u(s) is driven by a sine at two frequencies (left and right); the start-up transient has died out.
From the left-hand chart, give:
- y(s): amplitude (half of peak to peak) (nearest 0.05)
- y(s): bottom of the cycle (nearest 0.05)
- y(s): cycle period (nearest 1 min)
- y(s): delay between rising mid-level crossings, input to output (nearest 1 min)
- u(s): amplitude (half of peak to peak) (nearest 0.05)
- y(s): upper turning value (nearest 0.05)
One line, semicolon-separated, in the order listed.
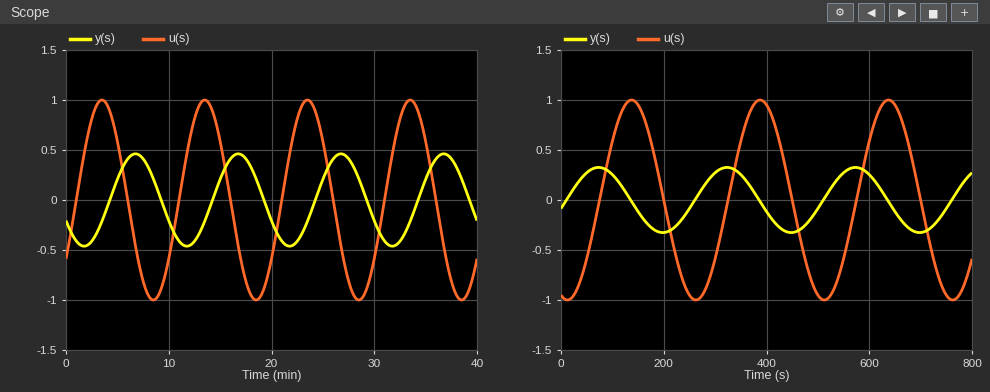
0.45; -0.45; 10 min; 3 min; 1.00; 0.45
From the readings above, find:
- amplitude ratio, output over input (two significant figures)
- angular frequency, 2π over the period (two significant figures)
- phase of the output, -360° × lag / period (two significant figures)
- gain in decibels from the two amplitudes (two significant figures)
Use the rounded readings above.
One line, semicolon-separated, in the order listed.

0.45; 0.63 rad/min; -110°; -6.9 dB
